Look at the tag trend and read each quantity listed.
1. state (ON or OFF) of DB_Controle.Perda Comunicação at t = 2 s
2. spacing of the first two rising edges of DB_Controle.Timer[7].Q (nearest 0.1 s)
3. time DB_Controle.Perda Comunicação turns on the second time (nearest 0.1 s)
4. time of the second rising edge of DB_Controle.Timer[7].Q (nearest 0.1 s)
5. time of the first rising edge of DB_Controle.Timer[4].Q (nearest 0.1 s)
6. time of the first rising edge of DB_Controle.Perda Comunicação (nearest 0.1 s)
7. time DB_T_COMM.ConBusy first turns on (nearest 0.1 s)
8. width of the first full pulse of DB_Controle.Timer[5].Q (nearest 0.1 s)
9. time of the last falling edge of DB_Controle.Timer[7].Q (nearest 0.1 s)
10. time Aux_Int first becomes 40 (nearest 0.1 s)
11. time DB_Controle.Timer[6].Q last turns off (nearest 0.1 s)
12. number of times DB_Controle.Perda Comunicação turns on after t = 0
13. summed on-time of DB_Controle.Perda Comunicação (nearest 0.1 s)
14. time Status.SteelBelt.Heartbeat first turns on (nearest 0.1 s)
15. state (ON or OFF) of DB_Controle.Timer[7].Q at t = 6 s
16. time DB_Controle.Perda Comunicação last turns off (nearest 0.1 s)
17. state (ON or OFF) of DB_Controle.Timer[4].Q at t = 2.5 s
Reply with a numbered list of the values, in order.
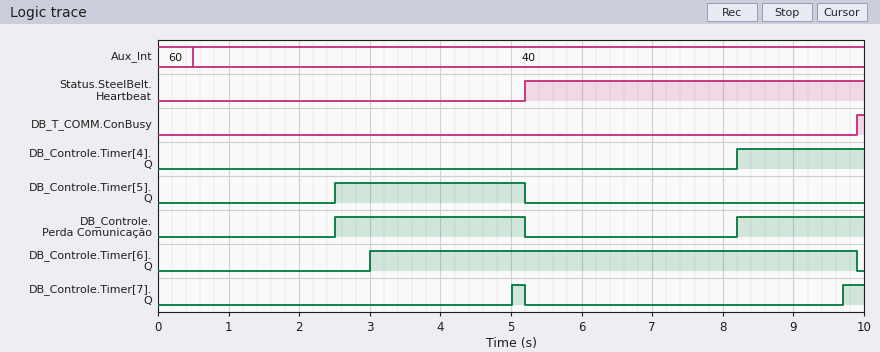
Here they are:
1. OFF
2. 4.7 s
3. 8.2 s
4. 9.7 s
5. 8.2 s
6. 2.5 s
7. 9.9 s
8. 2.7 s
9. 5.2 s
10. 0.5 s
11. 9.9 s
12. 2
13. 4.5 s
14. 5.2 s
15. OFF
16. 5.2 s
17. OFF
